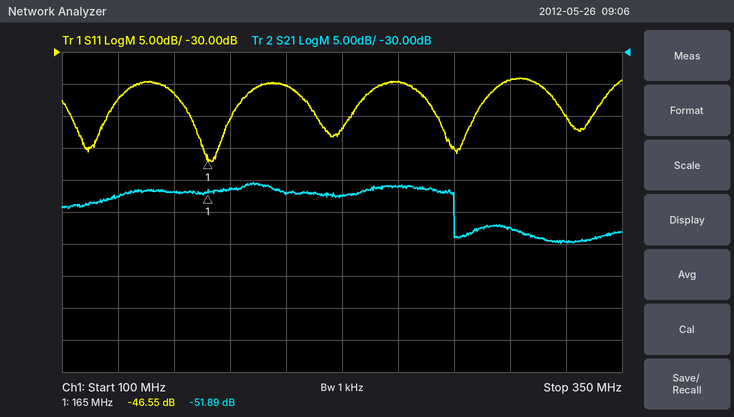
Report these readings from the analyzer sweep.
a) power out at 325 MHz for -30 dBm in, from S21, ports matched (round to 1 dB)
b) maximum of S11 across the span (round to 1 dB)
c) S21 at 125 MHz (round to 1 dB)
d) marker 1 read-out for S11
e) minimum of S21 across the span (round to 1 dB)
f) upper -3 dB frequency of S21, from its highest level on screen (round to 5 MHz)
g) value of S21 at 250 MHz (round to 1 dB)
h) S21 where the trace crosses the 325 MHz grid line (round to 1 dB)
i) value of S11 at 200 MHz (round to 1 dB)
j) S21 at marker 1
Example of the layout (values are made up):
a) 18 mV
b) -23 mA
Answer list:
a) -90 dBm
b) -34 dB
c) -53 dB
d) -46.55 dB
e) -60 dB
f) 275 MHz
g) -51 dB
h) -60 dB
i) -35 dB
j) -51.89 dB
